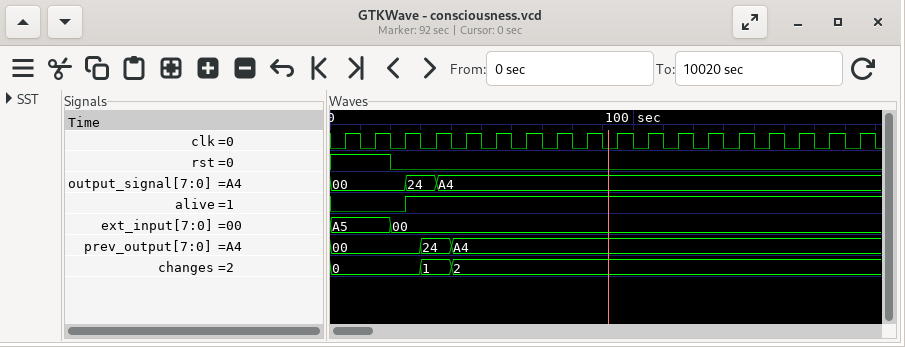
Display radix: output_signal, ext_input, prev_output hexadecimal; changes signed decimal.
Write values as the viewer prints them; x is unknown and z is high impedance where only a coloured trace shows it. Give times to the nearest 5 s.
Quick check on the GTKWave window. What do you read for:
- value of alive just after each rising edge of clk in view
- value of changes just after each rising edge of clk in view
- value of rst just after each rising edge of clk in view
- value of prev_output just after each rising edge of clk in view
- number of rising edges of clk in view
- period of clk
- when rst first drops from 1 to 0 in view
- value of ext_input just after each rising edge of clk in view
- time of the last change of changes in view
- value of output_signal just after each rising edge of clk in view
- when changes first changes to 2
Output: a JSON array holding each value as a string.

["0 0 1 1 1 1 1 1 1 1 1 1 1 1 1 1 1 1", "0, 0, 0, 1, 2, 2, 2, 2, 2, 2, 2, 2, 2, 2, 2, 2, 2, 2", "1 1 0 0 0 0 0 0 0 0 0 0 0 0 0 0 0 0", "00, 00, 00, 24, A4, A4, A4, A4, A4, A4, A4, A4, A4, A4, A4, A4, A4, A4", "18", "10 s", "20 s", "A5, A5, 00, 00, 00, 00, 00, 00, 00, 00, 00, 00, 00, 00, 00, 00, 00, 00", "40 s", "00, 00, 24, A4, A4, A4, A4, A4, A4, A4, A4, A4, A4, A4, A4, A4, A4, A4", "40 s"]
